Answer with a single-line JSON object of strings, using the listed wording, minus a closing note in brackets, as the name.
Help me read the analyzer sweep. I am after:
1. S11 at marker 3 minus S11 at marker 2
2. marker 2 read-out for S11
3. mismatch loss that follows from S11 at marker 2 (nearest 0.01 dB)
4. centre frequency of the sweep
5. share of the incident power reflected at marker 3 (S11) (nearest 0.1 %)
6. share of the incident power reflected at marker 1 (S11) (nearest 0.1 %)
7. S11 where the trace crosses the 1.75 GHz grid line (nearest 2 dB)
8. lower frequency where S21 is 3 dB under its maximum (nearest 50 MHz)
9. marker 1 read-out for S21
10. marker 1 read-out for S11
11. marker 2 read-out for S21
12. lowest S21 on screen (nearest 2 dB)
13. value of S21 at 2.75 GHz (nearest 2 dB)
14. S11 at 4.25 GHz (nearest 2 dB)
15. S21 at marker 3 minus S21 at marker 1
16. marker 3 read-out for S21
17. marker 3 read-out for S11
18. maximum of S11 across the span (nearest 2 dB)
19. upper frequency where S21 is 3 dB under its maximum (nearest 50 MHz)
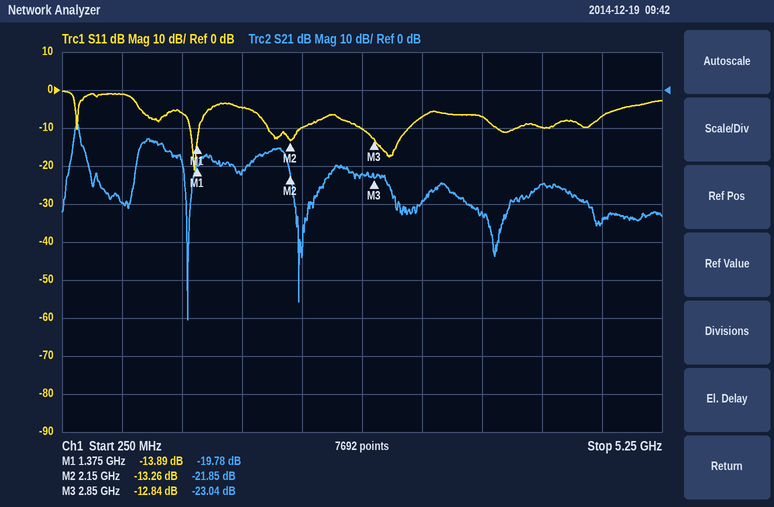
{"S11 at marker 3 minus S11 at marker 2": "0.42 dB", "marker 2 read-out for S11": "-13.26 dB", "mismatch loss that follows from S11 at marker 2": "0.21 dB", "centre frequency of the sweep": "2.75 GHz", "share of the incident power reflected at marker 3 (S11)": "5.2 %", "share of the incident power reflected at marker 1 (S11)": "4.1 %", "S11 where the trace crosses the 1.75 GHz grid line": "-4 dB", "lower frequency where S21 is 3 dB under its maximum": "350 MHz", "marker 1 read-out for S21": "-19.78 dB", "marker 1 read-out for S11": "-13.89 dB", "marker 2 read-out for S21": "-21.85 dB", "lowest S21 on screen": "-60 dB", "value of S21 at 2.75 GHz": "-22 dB", "S11 at 4.25 GHz": "-10 dB", "S21 at marker 3 minus S21 at marker 1": "-3.26 dB", "marker 3 read-out for S21": "-23.04 dB", "marker 3 read-out for S11": "-12.84 dB", "maximum of S11 across the span": "0 dB", "upper frequency where S21 is 3 dB under its maximum": "400 MHz"}
